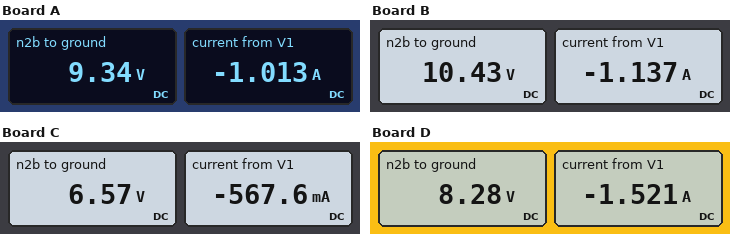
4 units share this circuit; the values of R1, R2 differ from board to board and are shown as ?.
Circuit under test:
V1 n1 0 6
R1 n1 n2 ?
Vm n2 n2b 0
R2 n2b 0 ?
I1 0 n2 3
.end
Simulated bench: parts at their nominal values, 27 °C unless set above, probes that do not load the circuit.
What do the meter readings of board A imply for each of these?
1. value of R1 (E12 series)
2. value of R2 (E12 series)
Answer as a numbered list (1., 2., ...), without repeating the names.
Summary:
1. 3.3 Ω
2. 4.7 Ω
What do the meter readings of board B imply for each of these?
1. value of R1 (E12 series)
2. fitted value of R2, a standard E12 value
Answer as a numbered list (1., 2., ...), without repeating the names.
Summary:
1. 3.9 Ω
2. 5.6 Ω
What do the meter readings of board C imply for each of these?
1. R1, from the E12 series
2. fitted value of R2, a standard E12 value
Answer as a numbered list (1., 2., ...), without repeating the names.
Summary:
1. 1 Ω
2. 2.7 Ω
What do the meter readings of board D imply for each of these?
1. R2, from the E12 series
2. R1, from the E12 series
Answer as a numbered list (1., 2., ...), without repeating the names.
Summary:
1. 5.6 Ω
2. 1.5 Ω
